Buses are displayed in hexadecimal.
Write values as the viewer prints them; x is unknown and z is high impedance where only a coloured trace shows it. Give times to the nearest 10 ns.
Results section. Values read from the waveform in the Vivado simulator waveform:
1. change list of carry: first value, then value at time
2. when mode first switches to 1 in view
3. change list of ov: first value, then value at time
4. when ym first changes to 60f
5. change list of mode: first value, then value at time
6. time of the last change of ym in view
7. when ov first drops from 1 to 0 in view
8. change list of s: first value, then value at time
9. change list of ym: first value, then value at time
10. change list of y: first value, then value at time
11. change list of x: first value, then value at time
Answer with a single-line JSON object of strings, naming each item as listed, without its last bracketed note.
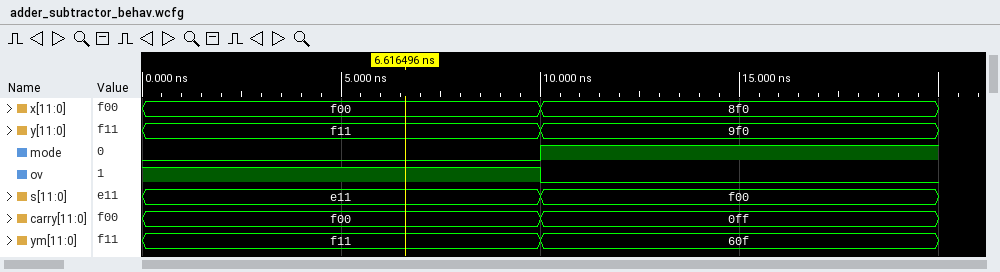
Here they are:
{"change list of carry: first value, then value at time": "f00, 0ff at 10 ns", "when mode first switches to 1 in view": "10 ns", "change list of ov: first value, then value at time": "1, 0 at 10 ns", "when ym first changes to 60f": "10 ns", "change list of mode: first value, then value at time": "0, 1 at 10 ns", "time of the last change of ym in view": "10 ns", "when ov first drops from 1 to 0 in view": "10 ns", "change list of s: first value, then value at time": "e11, f00 at 10 ns", "change list of ym: first value, then value at time": "f11, 60f at 10 ns", "change list of y: first value, then value at time": "f11, 9f0 at 10 ns", "change list of x: first value, then value at time": "f00, 8f0 at 10 ns"}
